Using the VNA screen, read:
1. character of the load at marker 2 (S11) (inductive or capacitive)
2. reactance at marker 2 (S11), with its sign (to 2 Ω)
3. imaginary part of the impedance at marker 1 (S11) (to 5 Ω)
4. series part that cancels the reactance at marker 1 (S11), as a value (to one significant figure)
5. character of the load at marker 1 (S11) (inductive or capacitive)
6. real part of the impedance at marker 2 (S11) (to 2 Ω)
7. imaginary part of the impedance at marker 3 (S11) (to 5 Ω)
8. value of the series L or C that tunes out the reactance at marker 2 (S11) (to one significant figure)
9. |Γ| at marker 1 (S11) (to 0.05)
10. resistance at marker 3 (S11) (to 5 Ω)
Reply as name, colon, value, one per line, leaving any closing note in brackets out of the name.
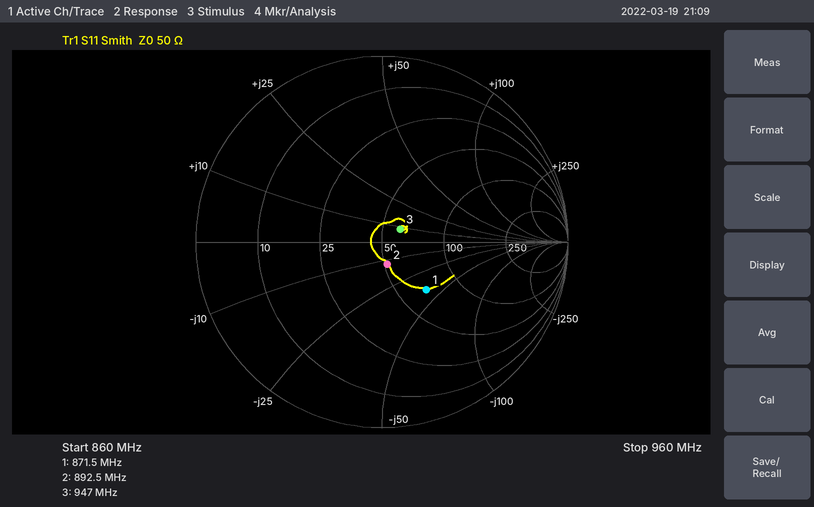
character of the load at marker 2 (S11): capacitive
reactance at marker 2 (S11), with its sign: -12 Ω
imaginary part of the impedance at marker 1 (S11): -40 Ω
series part that cancels the reactance at marker 1 (S11), as a value: 7 nH
character of the load at marker 1 (S11): capacitive
real part of the impedance at marker 2 (S11): 52 Ω
imaginary part of the impedance at marker 3 (S11): +10 Ω
value of the series L or C that tunes out the reactance at marker 2 (S11): 2 nH
|Γ| at marker 1 (S11): 0.35
resistance at marker 3 (S11): 60 Ω
